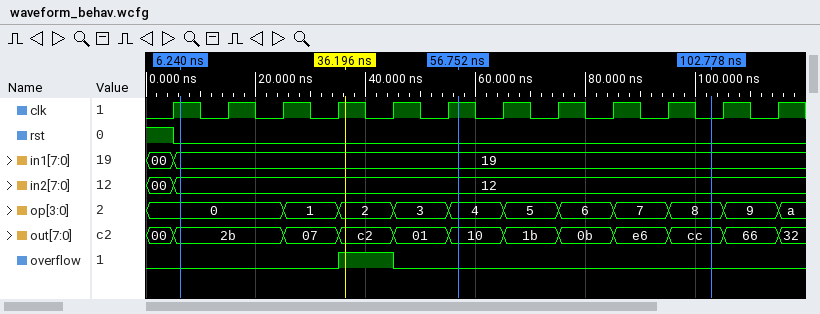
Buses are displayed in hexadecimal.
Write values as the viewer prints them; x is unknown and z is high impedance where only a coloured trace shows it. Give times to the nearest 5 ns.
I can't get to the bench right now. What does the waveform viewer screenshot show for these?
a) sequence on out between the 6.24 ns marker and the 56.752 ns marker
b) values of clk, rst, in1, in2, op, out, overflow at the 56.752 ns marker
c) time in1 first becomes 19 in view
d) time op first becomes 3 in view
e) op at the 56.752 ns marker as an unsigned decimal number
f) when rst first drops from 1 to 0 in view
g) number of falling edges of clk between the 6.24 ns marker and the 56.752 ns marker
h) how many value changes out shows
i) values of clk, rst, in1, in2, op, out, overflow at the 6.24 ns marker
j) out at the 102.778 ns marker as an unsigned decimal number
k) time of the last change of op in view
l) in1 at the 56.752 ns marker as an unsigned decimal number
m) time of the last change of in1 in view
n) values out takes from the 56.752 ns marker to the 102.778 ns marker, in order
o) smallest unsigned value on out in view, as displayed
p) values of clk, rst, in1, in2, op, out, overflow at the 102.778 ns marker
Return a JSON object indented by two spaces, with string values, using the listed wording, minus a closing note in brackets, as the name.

{
  "sequence on out between the 6.24 ns marker and the 56.752 ns marker": "2b, 07, c2, 01, 10",
  "values of clk, rst, in1, in2, op, out, overflow at the 56.752 ns marker": "clk=1, rst=0, in1=19, in2=12, op=4, out=10, overflow=0",
  "time in1 first becomes 19 in view": "5 ns",
  "time op first becomes 3 in view": "45 ns",
  "op at the 56.752 ns marker as an unsigned decimal number": "4",
  "when rst first drops from 1 to 0 in view": "5 ns",
  "number of falling edges of clk between the 6.24 ns marker and the 56.752 ns marker": "5",
  "how many value changes out shows": "11",
  "values of clk, rst, in1, in2, op, out, overflow at the 6.24 ns marker": "clk=1, rst=0, in1=19, in2=12, op=0, out=2b, overflow=0",
  "out at the 102.778 ns marker as an unsigned decimal number": "204",
  "time of the last change of op in view": "115 ns",
  "in1 at the 56.752 ns marker as an unsigned decimal number": "25",
  "time of the last change of in1 in view": "5 ns",
  "values out takes from the 56.752 ns marker to the 102.778 ns marker, in order": "10, 1b, 0b, e6, cc",
  "smallest unsigned value on out in view, as displayed": "00",
  "values of clk, rst, in1, in2, op, out, overflow at the 102.778 ns marker": "clk=0, rst=0, in1=19, in2=12, op=8, out=cc, overflow=0"
}
